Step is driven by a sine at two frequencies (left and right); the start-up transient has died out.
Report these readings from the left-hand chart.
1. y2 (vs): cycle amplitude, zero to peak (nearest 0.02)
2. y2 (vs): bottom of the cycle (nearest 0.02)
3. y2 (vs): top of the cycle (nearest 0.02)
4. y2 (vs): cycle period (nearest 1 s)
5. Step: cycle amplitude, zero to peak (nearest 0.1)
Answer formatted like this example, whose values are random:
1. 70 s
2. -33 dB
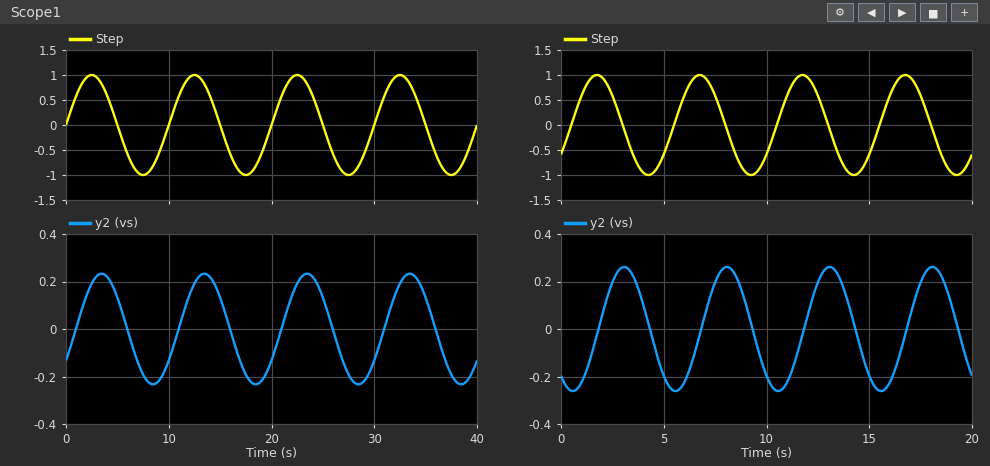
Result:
1. 0.24
2. -0.24
3. 0.24
4. 10 s
5. 1.0
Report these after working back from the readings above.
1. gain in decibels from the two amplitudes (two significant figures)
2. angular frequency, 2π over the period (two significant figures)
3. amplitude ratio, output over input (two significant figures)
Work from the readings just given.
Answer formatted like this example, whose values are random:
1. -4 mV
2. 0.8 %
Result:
1. -12 dB
2. 0.63 rad/s
3. 0.24
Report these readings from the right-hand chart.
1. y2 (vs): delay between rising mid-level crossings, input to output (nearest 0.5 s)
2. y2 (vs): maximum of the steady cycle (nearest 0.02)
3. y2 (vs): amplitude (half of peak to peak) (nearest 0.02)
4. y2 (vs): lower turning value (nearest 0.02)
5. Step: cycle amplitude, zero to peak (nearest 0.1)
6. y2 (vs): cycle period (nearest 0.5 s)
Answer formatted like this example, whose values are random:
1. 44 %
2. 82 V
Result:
1. 1.5 s
2. 0.26
3. 0.26
4. -0.26
5. 1.0
6. 5.0 s
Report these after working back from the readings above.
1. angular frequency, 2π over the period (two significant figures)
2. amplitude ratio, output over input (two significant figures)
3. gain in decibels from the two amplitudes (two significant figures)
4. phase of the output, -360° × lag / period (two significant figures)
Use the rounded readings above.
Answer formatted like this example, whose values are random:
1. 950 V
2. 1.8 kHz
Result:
1. 1.3 rad/s
2. 0.26
3. -12 dB
4. -110°
